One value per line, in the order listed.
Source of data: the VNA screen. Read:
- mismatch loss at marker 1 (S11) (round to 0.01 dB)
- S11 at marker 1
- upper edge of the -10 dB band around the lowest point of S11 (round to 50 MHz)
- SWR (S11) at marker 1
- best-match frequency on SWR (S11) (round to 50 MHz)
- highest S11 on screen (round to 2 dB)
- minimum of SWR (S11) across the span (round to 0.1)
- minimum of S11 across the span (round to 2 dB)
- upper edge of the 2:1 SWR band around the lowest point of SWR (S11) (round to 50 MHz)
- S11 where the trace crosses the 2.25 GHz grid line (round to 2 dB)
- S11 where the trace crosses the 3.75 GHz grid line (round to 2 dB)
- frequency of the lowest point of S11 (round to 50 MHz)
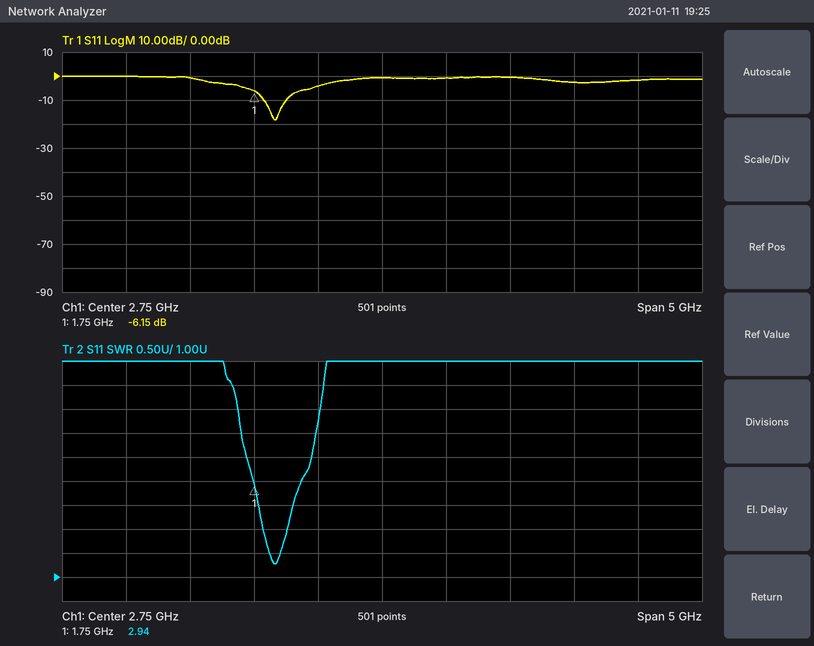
1.21 dB
-6.15 dB
2.00 GHz
2.94
1.90 GHz
0 dB
1.3
-18 dB
2.00 GHz
-4 dB
0 dB
1.90 GHz
